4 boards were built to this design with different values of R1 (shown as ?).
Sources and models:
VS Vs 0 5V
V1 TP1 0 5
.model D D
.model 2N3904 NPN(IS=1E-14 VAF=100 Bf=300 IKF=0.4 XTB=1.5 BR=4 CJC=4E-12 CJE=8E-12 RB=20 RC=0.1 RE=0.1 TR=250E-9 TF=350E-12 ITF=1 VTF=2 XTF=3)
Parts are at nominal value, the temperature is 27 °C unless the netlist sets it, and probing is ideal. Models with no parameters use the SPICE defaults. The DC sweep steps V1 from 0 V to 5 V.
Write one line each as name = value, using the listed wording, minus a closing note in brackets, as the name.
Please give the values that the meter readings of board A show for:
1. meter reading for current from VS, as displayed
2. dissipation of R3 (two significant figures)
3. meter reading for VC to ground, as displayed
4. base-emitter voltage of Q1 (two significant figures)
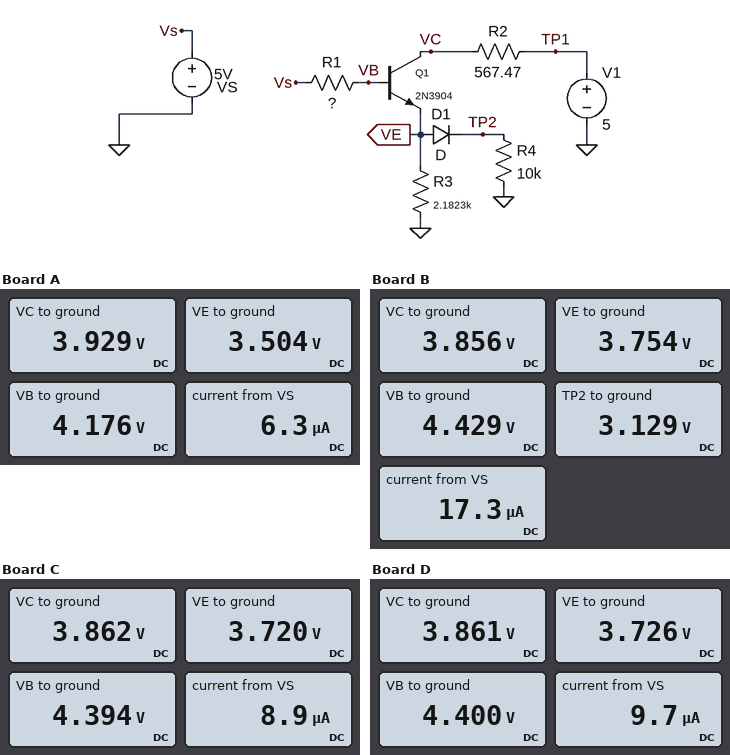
meter reading for current from VS, as displayed = 6.3 µA
dissipation of R3 = 5.6 mW
meter reading for VC to ground, as displayed = 3.929 V
base-emitter voltage of Q1 = 670 mV
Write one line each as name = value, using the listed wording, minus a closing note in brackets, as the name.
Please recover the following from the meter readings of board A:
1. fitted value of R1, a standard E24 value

fitted value of R1, a standard E24 value = 130 kΩ
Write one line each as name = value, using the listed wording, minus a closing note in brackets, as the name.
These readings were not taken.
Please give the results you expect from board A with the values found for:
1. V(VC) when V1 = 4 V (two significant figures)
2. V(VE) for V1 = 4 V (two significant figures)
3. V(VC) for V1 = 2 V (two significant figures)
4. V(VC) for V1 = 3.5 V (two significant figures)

V(VC) when V1 = 4 V = 3.1 V
V(VE) for V1 = 4 V = 3.0 V
V(VC) for V1 = 2 V = 1.6 V
V(VC) for V1 = 3.5 V = 2.7 V
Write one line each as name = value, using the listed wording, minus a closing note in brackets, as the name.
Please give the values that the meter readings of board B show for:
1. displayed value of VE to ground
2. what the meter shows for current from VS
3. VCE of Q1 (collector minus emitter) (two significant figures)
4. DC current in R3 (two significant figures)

displayed value of VE to ground = 3.754 V
what the meter shows for current from VS = 17.3 µA
VCE of Q1 (collector minus emitter) = 100 mV
DC current in R3 = 1.7 mA
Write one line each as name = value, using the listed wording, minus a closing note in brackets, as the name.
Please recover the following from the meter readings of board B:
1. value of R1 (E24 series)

value of R1 = 33 kΩ
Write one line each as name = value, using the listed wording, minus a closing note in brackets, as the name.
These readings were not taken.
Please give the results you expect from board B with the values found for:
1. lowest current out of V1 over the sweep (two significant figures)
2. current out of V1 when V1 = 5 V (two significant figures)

lowest current out of V1 over the sweep = -100 µA
current out of V1 when V1 = 5 V = 2.0 mA
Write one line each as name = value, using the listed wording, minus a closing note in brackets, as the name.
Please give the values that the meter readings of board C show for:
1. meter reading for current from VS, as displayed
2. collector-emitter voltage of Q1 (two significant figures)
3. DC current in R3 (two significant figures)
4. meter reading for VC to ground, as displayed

meter reading for current from VS, as displayed = 8.9 µA
collector-emitter voltage of Q1 = 140 mV
DC current in R3 = 1.7 mA
meter reading for VC to ground, as displayed = 3.862 V
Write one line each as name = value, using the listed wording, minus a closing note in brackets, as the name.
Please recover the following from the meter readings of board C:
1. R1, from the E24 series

R1, from the E24 series = 68 kΩ
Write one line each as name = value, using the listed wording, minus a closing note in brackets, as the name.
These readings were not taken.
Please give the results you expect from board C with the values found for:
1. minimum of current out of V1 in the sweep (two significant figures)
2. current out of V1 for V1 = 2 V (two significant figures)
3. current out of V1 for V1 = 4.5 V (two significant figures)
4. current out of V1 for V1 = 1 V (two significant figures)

minimum of current out of V1 in the sweep = -51 µA
current out of V1 for V1 = 2 V = 750 µA
current out of V1 for V1 = 4.5 V = 1.8 mA
current out of V1 for V1 = 1 V = 330 µA
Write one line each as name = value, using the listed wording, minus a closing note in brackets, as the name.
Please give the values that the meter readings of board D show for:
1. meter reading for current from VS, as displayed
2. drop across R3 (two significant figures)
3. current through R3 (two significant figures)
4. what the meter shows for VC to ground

meter reading for current from VS, as displayed = 9.7 µA
drop across R3 = 3.7 V
current through R3 = 1.7 mA
what the meter shows for VC to ground = 3.861 V
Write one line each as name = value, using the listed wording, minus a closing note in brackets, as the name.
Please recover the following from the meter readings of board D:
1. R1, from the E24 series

R1, from the E24 series = 62 kΩ
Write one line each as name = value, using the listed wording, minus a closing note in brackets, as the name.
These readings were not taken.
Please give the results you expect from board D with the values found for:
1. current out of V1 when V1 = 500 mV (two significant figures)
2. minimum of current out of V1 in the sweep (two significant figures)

current out of V1 when V1 = 500 mV = 130 µA
minimum of current out of V1 in the sweep = -56 µA
